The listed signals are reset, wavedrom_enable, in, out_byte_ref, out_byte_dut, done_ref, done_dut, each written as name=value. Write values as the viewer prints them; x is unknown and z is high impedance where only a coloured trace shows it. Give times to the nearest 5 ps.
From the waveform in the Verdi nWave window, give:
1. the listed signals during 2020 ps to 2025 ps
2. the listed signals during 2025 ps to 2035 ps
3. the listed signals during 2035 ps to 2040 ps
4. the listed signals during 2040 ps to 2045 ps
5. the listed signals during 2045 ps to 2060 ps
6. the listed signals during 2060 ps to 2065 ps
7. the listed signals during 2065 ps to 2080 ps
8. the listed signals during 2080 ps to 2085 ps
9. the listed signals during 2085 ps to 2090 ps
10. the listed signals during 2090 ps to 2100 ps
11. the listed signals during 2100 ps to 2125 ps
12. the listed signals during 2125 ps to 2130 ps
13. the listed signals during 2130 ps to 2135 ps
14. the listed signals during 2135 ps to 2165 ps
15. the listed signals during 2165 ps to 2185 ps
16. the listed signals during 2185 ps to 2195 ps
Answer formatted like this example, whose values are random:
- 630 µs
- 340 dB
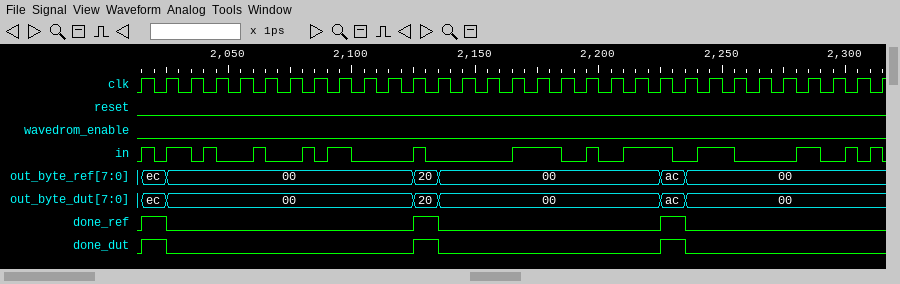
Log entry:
- reset=0, wavedrom_enable=0, in=0, out_byte_ref=ec, out_byte_dut=ec, done_ref=1, done_dut=1
- reset=0, wavedrom_enable=0, in=1, out_byte_ref=00, out_byte_dut=00, done_ref=0, done_dut=0
- reset=0, wavedrom_enable=0, in=0, out_byte_ref=00, out_byte_dut=00, done_ref=0, done_dut=0
- reset=0, wavedrom_enable=0, in=1, out_byte_ref=00, out_byte_dut=00, done_ref=0, done_dut=0
- reset=0, wavedrom_enable=0, in=0, out_byte_ref=00, out_byte_dut=00, done_ref=0, done_dut=0
- reset=0, wavedrom_enable=0, in=1, out_byte_ref=00, out_byte_dut=00, done_ref=0, done_dut=0
- reset=0, wavedrom_enable=0, in=0, out_byte_ref=00, out_byte_dut=00, done_ref=0, done_dut=0
- reset=0, wavedrom_enable=0, in=1, out_byte_ref=00, out_byte_dut=00, done_ref=0, done_dut=0
- reset=0, wavedrom_enable=0, in=0, out_byte_ref=00, out_byte_dut=00, done_ref=0, done_dut=0
- reset=0, wavedrom_enable=0, in=1, out_byte_ref=00, out_byte_dut=00, done_ref=0, done_dut=0
- reset=0, wavedrom_enable=0, in=0, out_byte_ref=00, out_byte_dut=00, done_ref=0, done_dut=0
- reset=0, wavedrom_enable=0, in=1, out_byte_ref=20, out_byte_dut=20, done_ref=1, done_dut=1
- reset=0, wavedrom_enable=0, in=0, out_byte_ref=20, out_byte_dut=20, done_ref=1, done_dut=1
- reset=0, wavedrom_enable=0, in=0, out_byte_ref=00, out_byte_dut=00, done_ref=0, done_dut=0
- reset=0, wavedrom_enable=0, in=1, out_byte_ref=00, out_byte_dut=00, done_ref=0, done_dut=0
- reset=0, wavedrom_enable=0, in=0, out_byte_ref=00, out_byte_dut=00, done_ref=0, done_dut=0
